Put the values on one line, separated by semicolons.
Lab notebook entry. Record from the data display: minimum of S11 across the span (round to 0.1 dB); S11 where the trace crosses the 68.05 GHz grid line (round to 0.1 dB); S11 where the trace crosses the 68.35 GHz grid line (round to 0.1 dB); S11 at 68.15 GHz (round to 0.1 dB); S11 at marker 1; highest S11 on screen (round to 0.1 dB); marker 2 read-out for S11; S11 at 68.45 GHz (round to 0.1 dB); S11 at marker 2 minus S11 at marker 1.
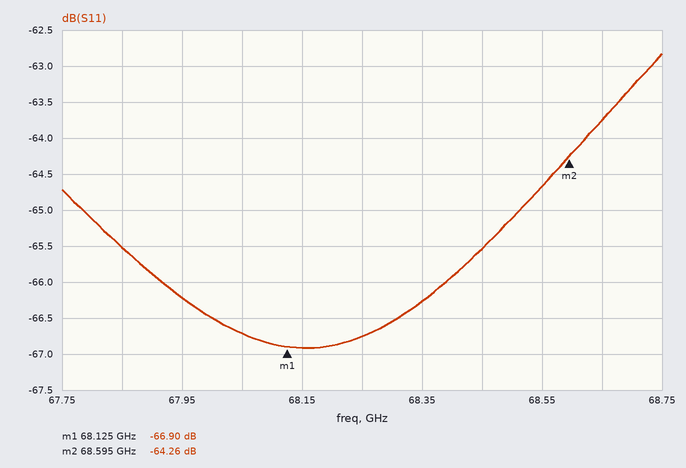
-66.9 dB; -66.7 dB; -66.3 dB; -66.9 dB; -66.90 dB; -62.8 dB; -64.26 dB; -65.5 dB; 2.64 dB
